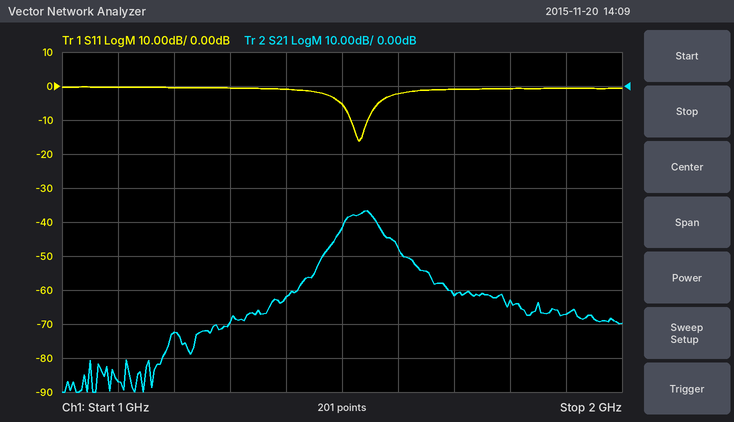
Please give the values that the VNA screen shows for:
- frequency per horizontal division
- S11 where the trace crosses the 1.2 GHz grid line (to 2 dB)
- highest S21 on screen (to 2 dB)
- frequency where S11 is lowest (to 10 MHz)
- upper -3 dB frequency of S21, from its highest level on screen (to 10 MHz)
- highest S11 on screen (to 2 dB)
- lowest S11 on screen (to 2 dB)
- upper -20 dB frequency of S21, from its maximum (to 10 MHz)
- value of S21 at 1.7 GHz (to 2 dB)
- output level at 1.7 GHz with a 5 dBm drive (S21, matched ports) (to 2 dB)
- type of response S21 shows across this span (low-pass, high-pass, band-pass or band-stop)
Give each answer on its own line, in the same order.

100 MHz
0 dB
-36 dB
1.53 GHz
1.56 GHz
0 dB
-16 dB
1.66 GHz
-62 dB
-56 dBm
band-pass
